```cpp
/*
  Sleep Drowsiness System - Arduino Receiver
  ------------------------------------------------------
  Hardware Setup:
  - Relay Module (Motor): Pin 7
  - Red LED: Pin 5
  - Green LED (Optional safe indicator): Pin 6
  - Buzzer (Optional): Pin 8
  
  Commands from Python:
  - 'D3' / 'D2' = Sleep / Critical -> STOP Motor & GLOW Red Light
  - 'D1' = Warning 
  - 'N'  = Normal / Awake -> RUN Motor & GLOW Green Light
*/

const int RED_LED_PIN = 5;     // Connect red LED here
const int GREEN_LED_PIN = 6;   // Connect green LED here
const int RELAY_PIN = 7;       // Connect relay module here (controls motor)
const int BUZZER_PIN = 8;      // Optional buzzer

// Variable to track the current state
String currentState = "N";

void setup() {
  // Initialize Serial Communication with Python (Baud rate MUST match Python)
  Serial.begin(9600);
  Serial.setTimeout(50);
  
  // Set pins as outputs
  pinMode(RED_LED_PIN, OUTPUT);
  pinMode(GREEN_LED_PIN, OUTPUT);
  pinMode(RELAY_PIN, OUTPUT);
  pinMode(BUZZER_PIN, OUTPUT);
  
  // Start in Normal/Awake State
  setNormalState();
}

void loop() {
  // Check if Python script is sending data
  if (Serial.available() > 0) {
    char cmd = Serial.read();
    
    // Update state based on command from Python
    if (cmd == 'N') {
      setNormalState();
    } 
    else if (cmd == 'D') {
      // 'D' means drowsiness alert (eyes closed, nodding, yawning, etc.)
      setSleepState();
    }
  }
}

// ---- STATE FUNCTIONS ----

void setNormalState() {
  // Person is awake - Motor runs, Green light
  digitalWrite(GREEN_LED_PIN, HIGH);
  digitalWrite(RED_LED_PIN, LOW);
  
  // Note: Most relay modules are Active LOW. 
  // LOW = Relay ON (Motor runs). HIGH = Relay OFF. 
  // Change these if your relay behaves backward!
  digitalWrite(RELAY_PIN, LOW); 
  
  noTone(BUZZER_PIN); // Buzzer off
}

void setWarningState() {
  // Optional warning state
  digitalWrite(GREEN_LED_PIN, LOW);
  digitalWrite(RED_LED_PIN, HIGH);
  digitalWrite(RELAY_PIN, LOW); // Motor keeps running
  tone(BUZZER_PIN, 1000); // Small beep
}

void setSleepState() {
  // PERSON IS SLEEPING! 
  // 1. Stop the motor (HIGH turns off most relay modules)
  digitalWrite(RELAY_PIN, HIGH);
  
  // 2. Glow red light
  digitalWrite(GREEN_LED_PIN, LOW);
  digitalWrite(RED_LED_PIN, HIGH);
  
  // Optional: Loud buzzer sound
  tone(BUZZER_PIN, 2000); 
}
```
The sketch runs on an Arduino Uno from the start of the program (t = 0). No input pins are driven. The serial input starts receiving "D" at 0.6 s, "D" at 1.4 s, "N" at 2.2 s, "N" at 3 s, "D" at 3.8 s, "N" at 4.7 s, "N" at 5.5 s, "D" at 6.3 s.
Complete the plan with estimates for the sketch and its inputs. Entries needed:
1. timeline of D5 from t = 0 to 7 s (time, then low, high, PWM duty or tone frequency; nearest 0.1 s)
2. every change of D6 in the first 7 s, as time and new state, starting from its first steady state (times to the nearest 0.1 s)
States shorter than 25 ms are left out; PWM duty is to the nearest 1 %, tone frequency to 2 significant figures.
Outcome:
0 s low; 0.6 s high; 2.2 s low; 3.8 s high; 4.7 s low; 6.3 s high
0 s high; 0.6 s low; 2.2 s high; 3.8 s low; 4.7 s high; 6.3 s low
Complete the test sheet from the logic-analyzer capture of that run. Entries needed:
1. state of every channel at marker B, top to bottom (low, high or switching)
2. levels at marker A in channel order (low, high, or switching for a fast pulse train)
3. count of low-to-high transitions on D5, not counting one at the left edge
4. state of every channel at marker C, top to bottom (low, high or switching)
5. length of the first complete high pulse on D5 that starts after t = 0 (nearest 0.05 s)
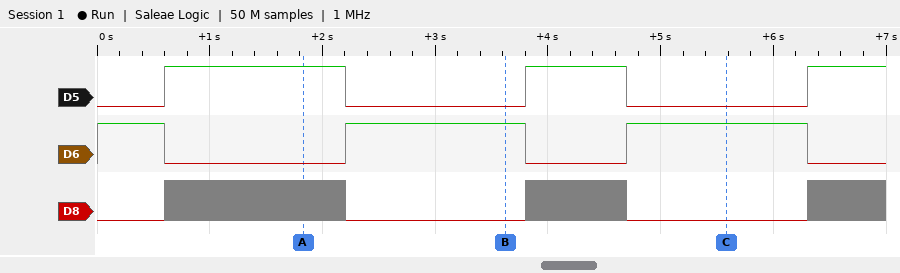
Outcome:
D5 low, D6 high, D8 low
D5 high, D6 low, D8 switching
3
D5 low, D6 high, D8 low
1.60 s
